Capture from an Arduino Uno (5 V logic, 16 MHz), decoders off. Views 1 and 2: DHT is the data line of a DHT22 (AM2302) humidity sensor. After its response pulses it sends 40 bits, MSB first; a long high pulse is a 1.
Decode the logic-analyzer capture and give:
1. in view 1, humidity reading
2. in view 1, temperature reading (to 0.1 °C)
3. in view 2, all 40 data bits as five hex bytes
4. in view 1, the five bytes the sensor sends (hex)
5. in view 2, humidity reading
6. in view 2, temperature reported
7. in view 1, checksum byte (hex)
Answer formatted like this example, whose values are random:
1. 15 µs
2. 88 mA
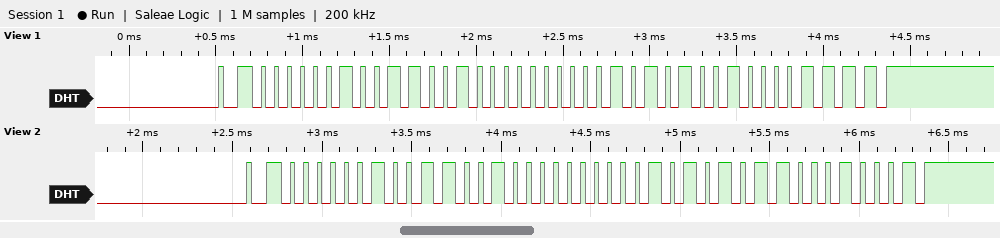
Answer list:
1. 61.2 %
2. 16.9 °C
3. 02 64 00 AB 11
4. 02 64 00 A9 0F
5. 61.2 %
6. 17.1 °C
7. 0x0F
